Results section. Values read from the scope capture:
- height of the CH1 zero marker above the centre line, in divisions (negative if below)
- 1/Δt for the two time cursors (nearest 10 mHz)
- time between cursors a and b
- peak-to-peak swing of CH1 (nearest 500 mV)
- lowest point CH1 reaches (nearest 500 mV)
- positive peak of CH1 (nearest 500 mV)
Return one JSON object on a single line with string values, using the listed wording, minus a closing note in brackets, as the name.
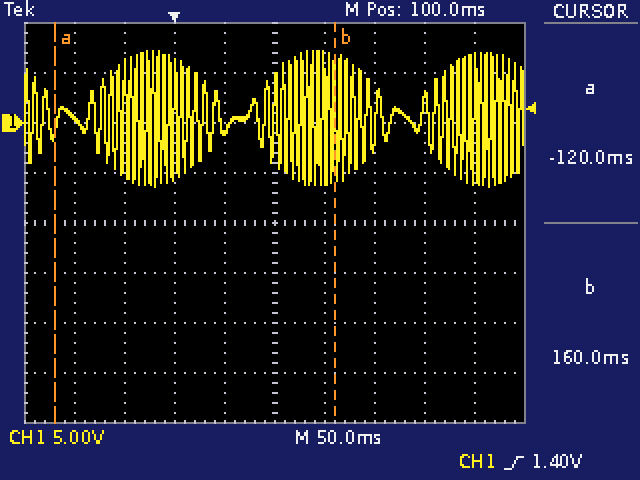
{"height of the CH1 zero marker above the centre line, in divisions": "+2.0 div", "1/Δt for the two time cursors": "3.57 Hz", "time between cursors a and b": "280 ms", "peak-to-peak swing of CH1": "13.5 V", "lowest point CH1 reaches": "-6.5 V", "positive peak of CH1": "7.0 V"}
